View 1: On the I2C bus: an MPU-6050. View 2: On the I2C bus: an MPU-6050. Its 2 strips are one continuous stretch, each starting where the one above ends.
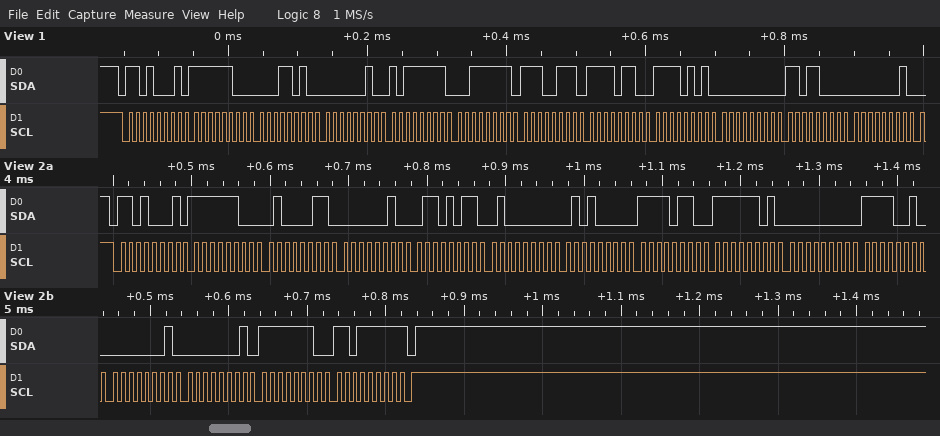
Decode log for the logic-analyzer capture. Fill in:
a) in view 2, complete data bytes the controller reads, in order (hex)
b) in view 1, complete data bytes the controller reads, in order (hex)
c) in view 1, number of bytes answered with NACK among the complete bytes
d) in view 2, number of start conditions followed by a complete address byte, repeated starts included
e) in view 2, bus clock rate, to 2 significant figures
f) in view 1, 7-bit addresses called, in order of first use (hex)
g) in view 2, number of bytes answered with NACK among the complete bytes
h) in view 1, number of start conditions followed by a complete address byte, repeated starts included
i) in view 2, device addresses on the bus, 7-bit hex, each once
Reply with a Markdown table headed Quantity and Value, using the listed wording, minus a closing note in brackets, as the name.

| Quantity | Value |
|---|---|
| in view 2, complete data bytes the controller reads, in order | FC 43 02 6B 40 50 F6 FD 00 F2 01 01 FE DF |
| in view 1, complete data bytes the controller reads, in order | FC 1A 02 BF 3F E7 F6 F5 00 D8 01 |
| in view 1, number of bytes answered with NACK among the complete bytes | 0 |
| in view 2, number of start conditions followed by a complete address byte, repeated starts included | 1 |
| in view 2, bus clock rate, to 2 significant figures | 100 kHz |
| in view 1, 7-bit addresses called, in order of first use | 0x68 |
| in view 2, number of bytes answered with NACK among the complete bytes | 1 |
| in view 1, number of start conditions followed by a complete address byte, repeated starts included | 1 |
| in view 2, device addresses on the bus, 7-bit hex, each once | 0x68 |
